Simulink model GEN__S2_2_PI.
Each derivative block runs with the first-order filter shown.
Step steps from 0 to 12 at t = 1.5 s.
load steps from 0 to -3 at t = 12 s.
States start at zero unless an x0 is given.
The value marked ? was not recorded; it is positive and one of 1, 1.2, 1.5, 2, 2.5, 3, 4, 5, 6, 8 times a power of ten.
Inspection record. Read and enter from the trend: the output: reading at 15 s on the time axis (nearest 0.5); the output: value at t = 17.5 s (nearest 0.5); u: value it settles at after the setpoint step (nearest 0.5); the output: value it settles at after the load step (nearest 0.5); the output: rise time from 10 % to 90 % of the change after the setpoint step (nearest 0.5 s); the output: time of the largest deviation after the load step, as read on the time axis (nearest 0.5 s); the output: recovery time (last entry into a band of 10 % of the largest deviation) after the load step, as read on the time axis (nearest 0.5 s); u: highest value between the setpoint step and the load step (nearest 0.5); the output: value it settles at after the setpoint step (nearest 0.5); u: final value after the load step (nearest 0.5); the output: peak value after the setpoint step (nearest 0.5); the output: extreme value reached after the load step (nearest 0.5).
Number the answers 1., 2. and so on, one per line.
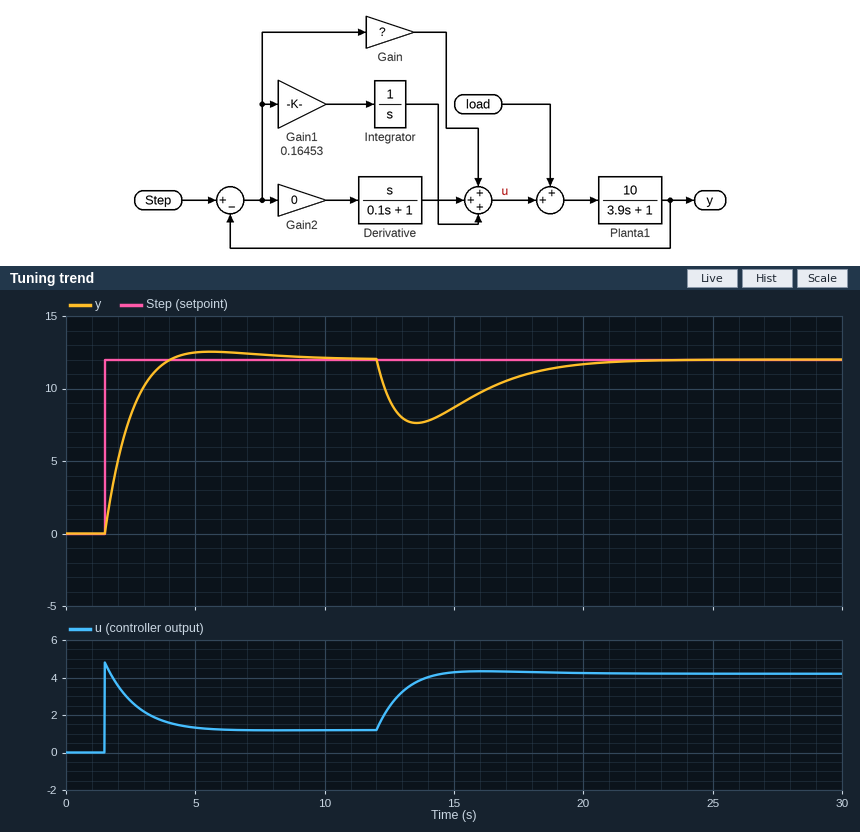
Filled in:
1. 8.5
2. 11.0
3. 1.0
4. 12.0
5. 1.5 s
6. 13.5 s
7. 19.5 s
8. 5.0
9. 12.0
10. 4.0
11. 12.5
12. 7.5
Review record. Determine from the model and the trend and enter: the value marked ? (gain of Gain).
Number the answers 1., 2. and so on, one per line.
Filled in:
1. 0.4
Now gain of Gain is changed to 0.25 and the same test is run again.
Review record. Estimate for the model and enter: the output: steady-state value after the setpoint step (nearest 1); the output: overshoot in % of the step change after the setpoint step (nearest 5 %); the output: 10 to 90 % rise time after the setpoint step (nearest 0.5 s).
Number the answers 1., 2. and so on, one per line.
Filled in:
1. 12
2. 10 %
3. 2.0 s
